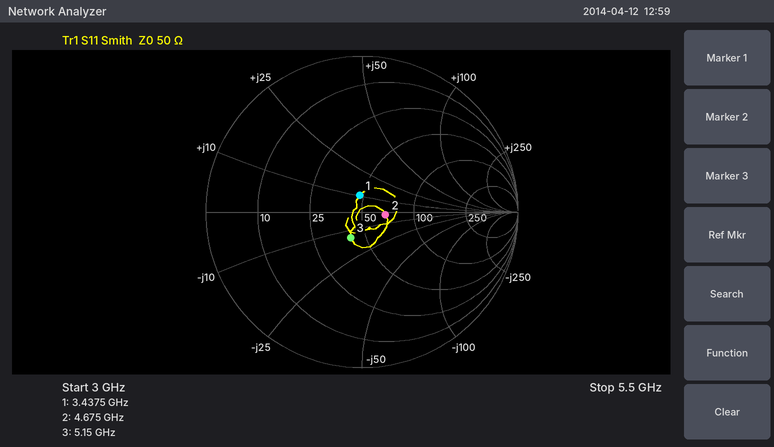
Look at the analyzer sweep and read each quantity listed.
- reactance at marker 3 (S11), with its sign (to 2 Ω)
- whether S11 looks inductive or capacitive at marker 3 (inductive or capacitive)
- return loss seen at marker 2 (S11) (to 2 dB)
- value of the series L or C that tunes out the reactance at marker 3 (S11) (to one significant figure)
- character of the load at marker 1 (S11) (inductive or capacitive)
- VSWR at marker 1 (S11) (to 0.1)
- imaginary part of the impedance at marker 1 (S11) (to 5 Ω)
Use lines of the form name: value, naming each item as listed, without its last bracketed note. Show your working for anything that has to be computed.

reactance at marker 3 (S11), with its sign: -14 Ω
whether S11 looks inductive or capacitive at marker 3: capacitive
return loss seen at marker 2 (S11): 16 dB
value of the series L or C that tunes out the reactance at marker 3 (S11): L = 14 Ω/(2π × 5.15 GHz) ≈ 433 pH, so 400 pH to one significant figure
character of the load at marker 1 (S11): inductive
VSWR at marker 1 (S11): 1.2
imaginary part of the impedance at marker 1 (S11): +10 Ω
